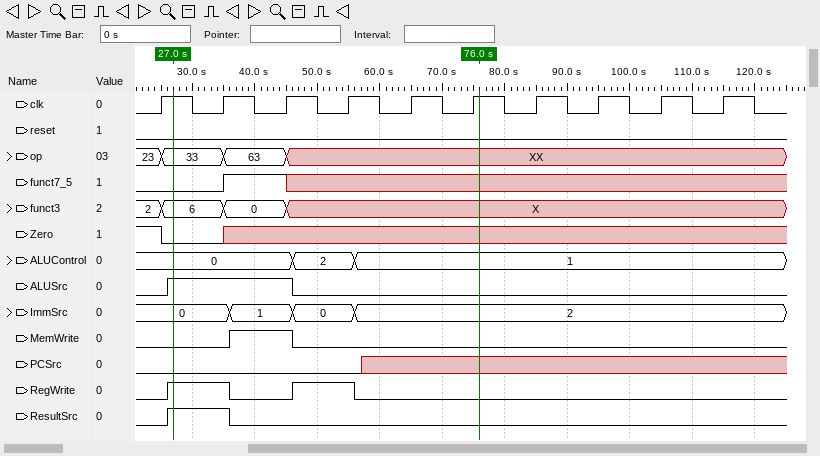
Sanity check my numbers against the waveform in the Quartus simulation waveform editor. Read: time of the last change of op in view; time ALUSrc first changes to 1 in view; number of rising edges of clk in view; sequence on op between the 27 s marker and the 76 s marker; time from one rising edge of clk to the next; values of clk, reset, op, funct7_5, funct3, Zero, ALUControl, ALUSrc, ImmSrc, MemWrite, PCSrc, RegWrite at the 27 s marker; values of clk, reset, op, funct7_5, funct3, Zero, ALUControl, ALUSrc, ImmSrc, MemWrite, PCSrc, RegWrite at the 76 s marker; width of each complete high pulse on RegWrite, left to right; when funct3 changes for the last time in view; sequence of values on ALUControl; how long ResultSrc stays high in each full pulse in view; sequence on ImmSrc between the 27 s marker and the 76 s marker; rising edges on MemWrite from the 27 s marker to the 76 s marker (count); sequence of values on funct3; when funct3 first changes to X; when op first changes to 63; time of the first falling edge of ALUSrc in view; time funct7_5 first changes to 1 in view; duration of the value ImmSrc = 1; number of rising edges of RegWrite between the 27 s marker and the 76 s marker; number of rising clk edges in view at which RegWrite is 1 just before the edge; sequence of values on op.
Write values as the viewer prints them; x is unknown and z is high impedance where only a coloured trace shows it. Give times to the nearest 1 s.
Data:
45 s
26 s
10
33, 63, XX
10 s
clk=1, reset=0, op=33, funct7_5=0, funct3=6, Zero=0, ALUControl=0, ALUSrc=1, ImmSrc=0, MemWrite=0, PCSrc=0, RegWrite=1
clk=1, reset=0, op=XX, funct7_5=x, funct3=X, Zero=x, ALUControl=1, ALUSrc=0, ImmSrc=2, MemWrite=0, PCSrc=x, RegWrite=0
10 s, 10 s
45 s
0, 2, 1
10 s
0, 1, 0, 2
1
2, 6, 0, X
45 s
35 s
46 s
35 s
10 s
1
2
23, 33, 63, XX
